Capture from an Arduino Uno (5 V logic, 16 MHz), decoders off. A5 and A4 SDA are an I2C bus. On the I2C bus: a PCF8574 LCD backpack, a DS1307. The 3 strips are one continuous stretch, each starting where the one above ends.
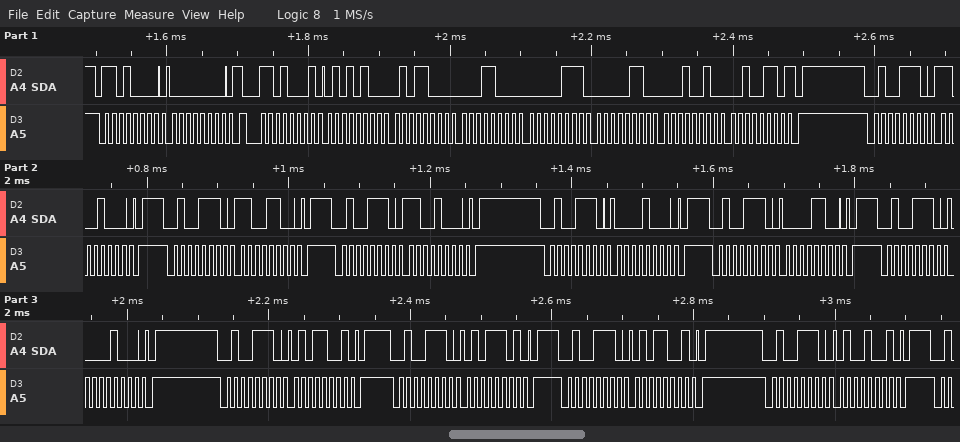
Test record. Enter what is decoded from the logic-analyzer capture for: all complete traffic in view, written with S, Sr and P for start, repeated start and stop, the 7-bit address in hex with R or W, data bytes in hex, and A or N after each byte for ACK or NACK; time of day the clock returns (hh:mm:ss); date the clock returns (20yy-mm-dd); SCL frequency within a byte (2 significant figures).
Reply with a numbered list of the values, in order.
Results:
1. S 68W A 00 A Sr 68R A 54 A 58 A 18 A 07 A 06 A 12 A 26 N P S 27W A C8 A P S 27W A CC A P S 27W A C8 A P S 27W A 08 A P S 27W A 0C A P S 27W A 08 A P S 27W A 59 A P S 27W A 5D A P S 27W A 59 A P S 27W A 49 A P
2. 18:58:54
3. 2026-12-06
4. 100 kHz
